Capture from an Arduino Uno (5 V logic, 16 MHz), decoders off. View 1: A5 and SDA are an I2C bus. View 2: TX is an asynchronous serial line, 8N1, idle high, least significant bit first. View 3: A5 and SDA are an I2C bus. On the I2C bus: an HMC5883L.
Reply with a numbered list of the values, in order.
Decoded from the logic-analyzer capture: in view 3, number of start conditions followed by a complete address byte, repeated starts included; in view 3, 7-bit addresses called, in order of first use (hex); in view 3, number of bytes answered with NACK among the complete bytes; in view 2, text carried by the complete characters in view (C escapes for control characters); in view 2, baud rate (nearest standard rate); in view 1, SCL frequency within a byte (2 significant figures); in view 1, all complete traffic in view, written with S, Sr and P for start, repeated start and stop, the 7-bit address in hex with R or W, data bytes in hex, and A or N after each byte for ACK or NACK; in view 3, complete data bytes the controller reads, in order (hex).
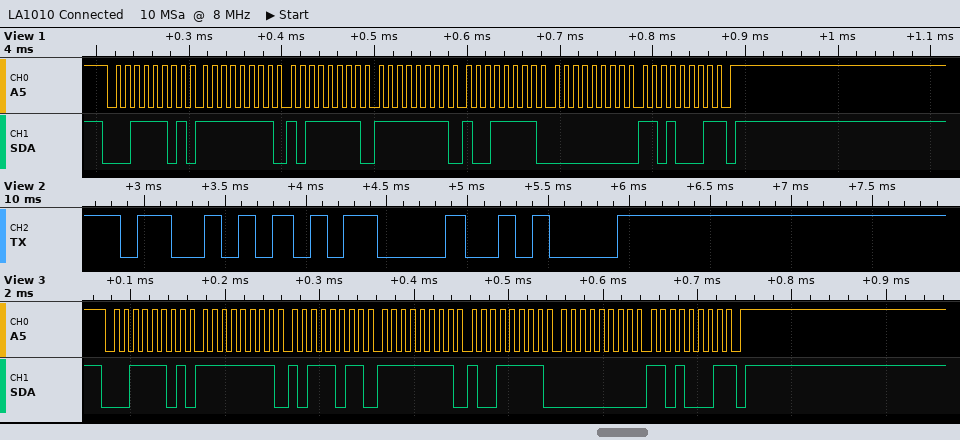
1. 1
2. 0x1E
3. 1
4. "S\r\n"
5. 9600 baud
6. 100 kHz
7. S 1ER A FF A BF A FF A 9F A 00 A D1 N P
8. FF BB FF 9F 00 D1
